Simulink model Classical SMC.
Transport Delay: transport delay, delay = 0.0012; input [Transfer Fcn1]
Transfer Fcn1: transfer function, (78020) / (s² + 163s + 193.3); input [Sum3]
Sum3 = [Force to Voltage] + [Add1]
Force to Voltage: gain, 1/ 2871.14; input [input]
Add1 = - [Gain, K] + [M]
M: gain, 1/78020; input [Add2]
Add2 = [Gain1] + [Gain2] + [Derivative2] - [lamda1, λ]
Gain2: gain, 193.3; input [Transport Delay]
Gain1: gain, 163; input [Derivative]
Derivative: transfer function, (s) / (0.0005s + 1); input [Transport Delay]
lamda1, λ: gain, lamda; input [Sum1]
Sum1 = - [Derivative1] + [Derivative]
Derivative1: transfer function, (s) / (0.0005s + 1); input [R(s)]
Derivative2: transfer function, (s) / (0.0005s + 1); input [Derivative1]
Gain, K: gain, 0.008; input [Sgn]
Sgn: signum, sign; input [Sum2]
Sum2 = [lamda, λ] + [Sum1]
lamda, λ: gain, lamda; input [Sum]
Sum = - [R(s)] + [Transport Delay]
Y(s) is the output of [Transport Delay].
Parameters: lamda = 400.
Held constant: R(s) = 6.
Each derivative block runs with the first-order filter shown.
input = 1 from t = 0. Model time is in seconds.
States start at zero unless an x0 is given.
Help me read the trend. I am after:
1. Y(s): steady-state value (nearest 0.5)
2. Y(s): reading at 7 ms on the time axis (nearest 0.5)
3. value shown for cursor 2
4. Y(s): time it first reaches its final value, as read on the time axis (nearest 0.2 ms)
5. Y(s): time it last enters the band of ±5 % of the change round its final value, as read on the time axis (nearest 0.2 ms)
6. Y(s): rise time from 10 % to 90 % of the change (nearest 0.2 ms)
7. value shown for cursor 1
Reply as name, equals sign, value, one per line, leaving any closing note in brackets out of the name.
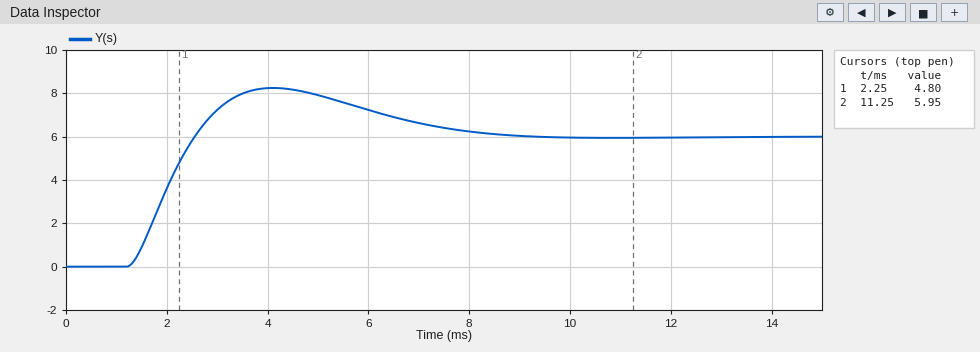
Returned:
Y(s): steady-state value = 6.0
Y(s): reading at 7 ms on the time axis = 6.5
value shown for cursor 2 = 5.95
Y(s): time it first reaches its final value, as read on the time axis = 2.6 ms
Y(s): time it last enters the band of ±5 % of the change round its final value, as read on the time axis = 7.8 ms
Y(s): rise time from 10 % to 90 % of the change = 1.0 ms
value shown for cursor 1 = 4.80
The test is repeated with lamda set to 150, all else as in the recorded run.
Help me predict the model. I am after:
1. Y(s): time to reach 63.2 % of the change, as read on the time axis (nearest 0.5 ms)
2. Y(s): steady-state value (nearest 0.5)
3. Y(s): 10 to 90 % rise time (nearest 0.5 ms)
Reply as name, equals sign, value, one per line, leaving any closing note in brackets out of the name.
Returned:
Y(s): time to reach 63.2 % of the change, as read on the time axis = 2.0 ms
Y(s): steady-state value = 6.0
Y(s): 10 to 90 % rise time = 1.5 ms
